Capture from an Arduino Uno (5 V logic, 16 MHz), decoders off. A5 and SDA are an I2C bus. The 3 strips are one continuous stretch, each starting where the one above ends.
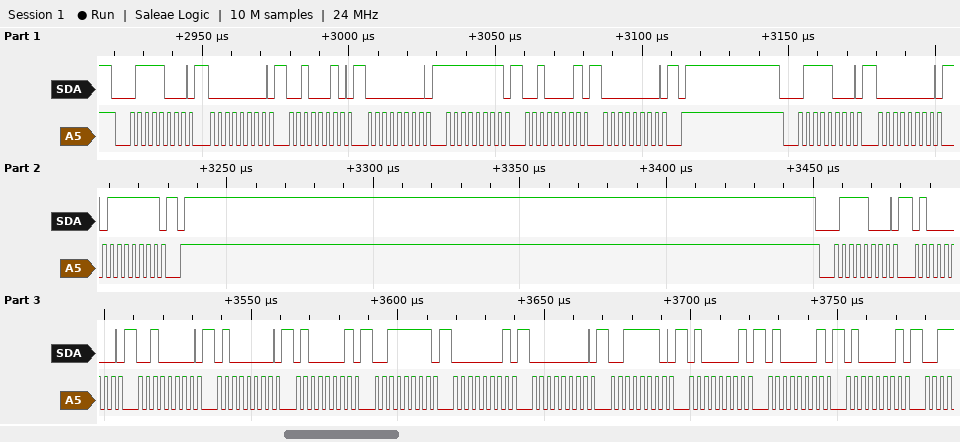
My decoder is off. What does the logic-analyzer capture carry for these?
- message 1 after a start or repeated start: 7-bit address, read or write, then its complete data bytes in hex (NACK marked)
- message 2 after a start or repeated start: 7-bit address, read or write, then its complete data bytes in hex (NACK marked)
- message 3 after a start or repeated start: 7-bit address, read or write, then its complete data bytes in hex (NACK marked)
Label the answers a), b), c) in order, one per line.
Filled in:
a) 0x3C write: 00 22 00 FF 21 00
b) 0x3C write: 00 7F
c) 0x3C write: 40 20 40 41 3F 01 00 3E 41 41 41
